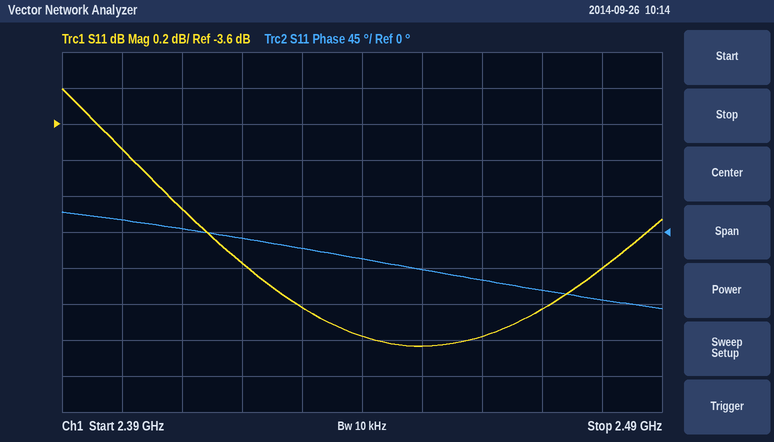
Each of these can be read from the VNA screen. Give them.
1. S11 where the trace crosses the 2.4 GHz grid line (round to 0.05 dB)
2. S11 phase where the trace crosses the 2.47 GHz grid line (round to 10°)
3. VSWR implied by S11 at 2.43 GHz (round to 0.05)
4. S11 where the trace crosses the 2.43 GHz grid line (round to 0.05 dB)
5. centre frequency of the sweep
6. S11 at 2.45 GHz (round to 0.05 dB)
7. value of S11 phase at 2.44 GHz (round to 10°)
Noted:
-3.75 dB
-70°
3.85
-4.60 dB
2.44 GHz
-4.85 dB
-30°
